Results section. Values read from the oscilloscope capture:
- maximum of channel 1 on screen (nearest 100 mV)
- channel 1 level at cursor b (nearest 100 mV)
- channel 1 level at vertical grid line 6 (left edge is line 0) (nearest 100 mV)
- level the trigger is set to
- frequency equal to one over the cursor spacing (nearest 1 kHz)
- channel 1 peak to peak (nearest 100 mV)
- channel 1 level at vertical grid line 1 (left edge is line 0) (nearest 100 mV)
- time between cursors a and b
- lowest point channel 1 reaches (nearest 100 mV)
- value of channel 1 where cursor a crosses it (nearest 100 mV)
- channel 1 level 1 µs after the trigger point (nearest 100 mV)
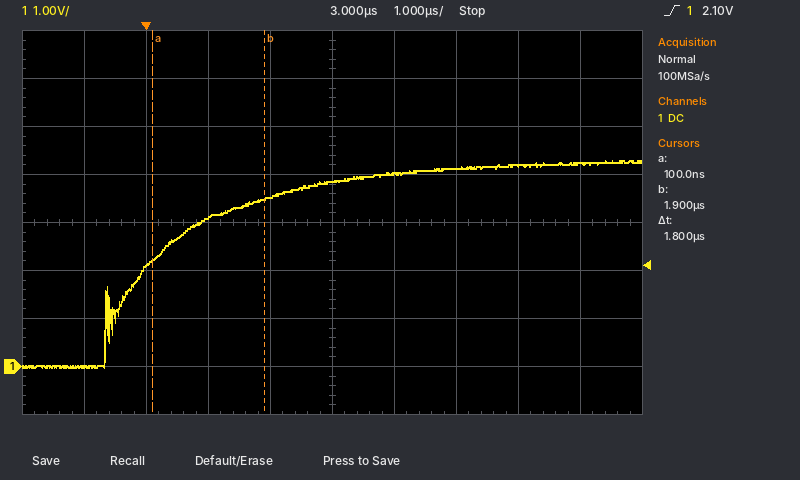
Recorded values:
4.3 V
3.5 V
4.0 V
2.10 V
556 kHz
4.3 V
0.0 V
1.8 µs
0.0 V
2.2 V
3.1 V
